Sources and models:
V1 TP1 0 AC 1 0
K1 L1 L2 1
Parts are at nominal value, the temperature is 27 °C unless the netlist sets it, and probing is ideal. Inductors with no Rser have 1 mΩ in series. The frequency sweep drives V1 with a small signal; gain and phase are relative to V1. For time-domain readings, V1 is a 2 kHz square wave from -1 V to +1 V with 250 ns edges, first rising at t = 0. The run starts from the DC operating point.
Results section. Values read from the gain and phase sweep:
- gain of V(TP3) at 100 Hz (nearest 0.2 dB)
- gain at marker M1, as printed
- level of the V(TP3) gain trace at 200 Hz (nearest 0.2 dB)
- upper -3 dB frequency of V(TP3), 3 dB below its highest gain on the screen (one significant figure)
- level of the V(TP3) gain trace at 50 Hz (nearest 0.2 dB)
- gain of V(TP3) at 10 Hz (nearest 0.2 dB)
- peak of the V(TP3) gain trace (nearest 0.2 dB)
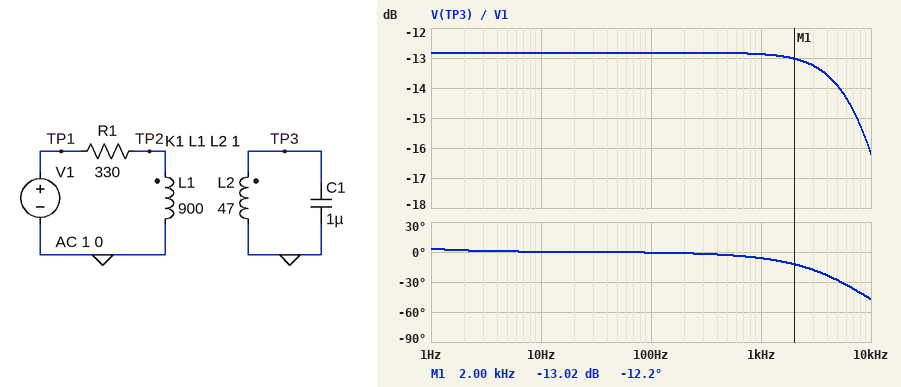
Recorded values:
-12.8 dB
-13.02 dB
-12.8 dB
9 kHz
-12.8 dB
-12.8 dB
-12.8 dB
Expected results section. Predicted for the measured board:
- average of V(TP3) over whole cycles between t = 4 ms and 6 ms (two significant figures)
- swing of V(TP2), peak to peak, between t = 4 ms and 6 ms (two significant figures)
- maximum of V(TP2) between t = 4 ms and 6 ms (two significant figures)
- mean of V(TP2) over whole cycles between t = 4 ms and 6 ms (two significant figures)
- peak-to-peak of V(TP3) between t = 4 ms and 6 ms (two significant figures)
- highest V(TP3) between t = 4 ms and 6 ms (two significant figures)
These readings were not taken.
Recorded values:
230 mV
2.0 V
2.0 V
1.0 V
460 mV
460 mV
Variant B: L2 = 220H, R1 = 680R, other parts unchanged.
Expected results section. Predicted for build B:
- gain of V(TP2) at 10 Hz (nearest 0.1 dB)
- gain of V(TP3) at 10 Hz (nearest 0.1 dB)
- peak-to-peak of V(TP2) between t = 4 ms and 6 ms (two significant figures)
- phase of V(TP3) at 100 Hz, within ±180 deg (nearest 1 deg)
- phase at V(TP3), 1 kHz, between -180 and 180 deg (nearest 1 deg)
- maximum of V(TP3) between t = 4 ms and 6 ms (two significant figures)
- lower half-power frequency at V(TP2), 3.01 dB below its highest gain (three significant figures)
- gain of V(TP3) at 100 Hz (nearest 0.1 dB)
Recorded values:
0 dB
-6.1 dB
1.3 V
-6 deg
-46 deg
810 mV
120 mHz
-6.2 dB
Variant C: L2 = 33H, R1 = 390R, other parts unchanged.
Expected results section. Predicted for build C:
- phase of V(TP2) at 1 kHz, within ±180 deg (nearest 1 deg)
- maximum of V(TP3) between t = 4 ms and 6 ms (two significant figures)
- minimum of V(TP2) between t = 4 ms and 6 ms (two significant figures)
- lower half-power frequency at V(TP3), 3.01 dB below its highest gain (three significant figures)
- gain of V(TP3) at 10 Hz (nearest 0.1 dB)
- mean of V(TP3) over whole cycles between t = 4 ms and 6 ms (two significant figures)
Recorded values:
-5 deg
380 mV
-2.6 mV
69.0 mHz
-14.4 dB
190 mV
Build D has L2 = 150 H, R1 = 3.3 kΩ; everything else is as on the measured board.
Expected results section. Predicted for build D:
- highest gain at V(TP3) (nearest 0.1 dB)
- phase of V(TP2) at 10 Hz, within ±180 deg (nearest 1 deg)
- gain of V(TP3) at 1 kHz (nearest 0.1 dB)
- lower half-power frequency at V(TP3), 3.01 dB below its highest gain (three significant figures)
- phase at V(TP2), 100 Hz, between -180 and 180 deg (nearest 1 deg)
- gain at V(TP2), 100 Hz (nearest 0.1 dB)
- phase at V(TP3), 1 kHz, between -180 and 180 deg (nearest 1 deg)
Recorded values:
-7.8 dB
1 deg
-18.9 dB
582 mHz
-19 deg
-0.5 dB
-74 deg
